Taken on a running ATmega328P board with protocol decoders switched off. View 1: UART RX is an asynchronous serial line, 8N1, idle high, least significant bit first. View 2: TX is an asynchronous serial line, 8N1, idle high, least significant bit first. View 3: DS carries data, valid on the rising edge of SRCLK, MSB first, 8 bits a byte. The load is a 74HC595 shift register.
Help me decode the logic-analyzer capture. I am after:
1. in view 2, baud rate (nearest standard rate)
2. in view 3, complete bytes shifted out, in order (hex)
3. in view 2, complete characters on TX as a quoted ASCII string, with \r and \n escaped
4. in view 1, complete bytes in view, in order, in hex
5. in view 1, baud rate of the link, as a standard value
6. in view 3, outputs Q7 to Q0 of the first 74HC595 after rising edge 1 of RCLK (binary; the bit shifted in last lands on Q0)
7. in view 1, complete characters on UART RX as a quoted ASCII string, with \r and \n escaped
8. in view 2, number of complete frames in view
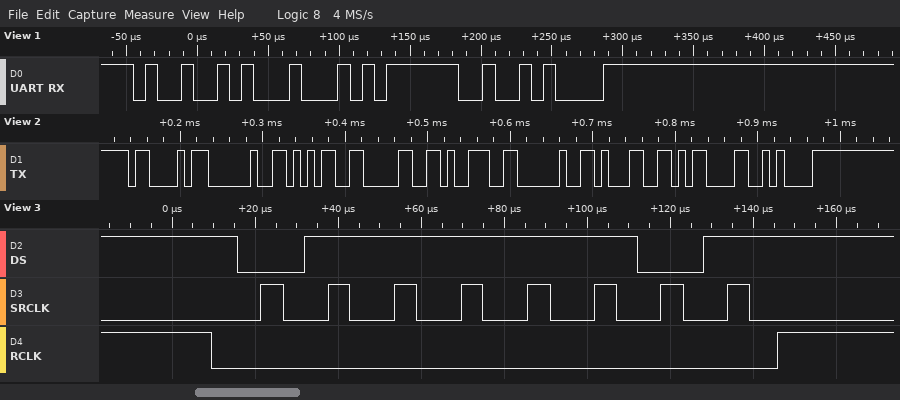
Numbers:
115200 baud
7D
"C 509 1\r\n"
0x49 0x44 0x3F 0x0A
115200 baud
01111101
"ID?\n"
9
